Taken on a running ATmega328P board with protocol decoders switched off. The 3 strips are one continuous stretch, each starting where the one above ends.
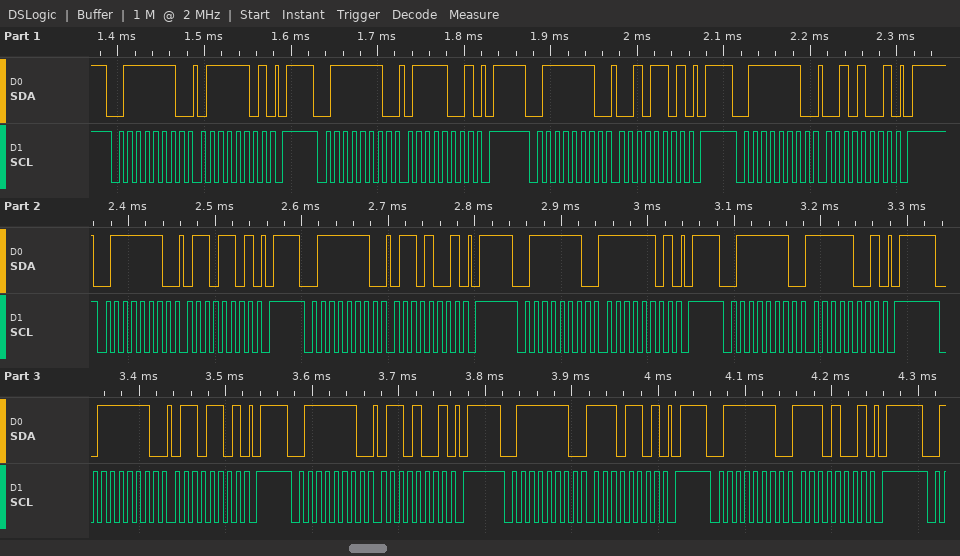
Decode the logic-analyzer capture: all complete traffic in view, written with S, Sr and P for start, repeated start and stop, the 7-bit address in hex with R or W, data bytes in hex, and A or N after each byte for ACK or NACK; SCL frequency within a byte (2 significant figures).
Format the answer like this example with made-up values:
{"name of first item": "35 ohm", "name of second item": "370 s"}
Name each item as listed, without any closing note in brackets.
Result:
{"all complete traffic in view, written with S, Sr and P for start, repeated start and stop, the 7-bit address in hex with R or W, data bytes in hex, and A or N after each byte for ACK or NACK": "S 3FW A 7D A P S 3FW A 79 A P S 3FW A 2D A P S 3FW A 29 A P S 3FW A 6D A P S 3FW A 69 A P S 3FW A FD A P S 3FW A F9 A P S 3FW A 6D A P S 3FW A 69 A P S 3FW A ED A P S 3FW A E9 A P", "SCL frequency within a byte": "100 kHz"}
